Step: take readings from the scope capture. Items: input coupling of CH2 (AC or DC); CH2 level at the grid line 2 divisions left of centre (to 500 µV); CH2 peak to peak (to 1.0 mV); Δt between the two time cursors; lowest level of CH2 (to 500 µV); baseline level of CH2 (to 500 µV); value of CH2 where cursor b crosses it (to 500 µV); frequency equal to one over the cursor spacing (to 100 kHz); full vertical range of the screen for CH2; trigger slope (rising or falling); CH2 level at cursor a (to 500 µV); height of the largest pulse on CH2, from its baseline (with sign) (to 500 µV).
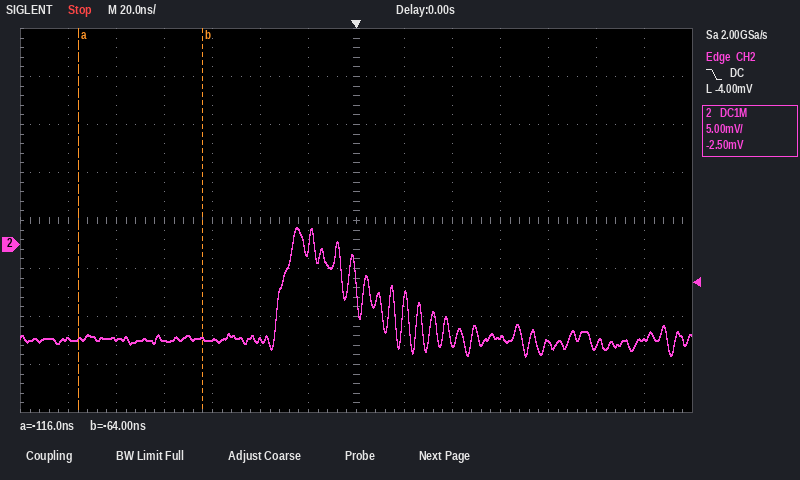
DC
-10.0 mV
13.0 mV
52 ns
-11.5 mV
-10.0 mV
-10.0 mV
19.2 MHz
40 mV
falling
-10.0 mV
+11.5 mV
